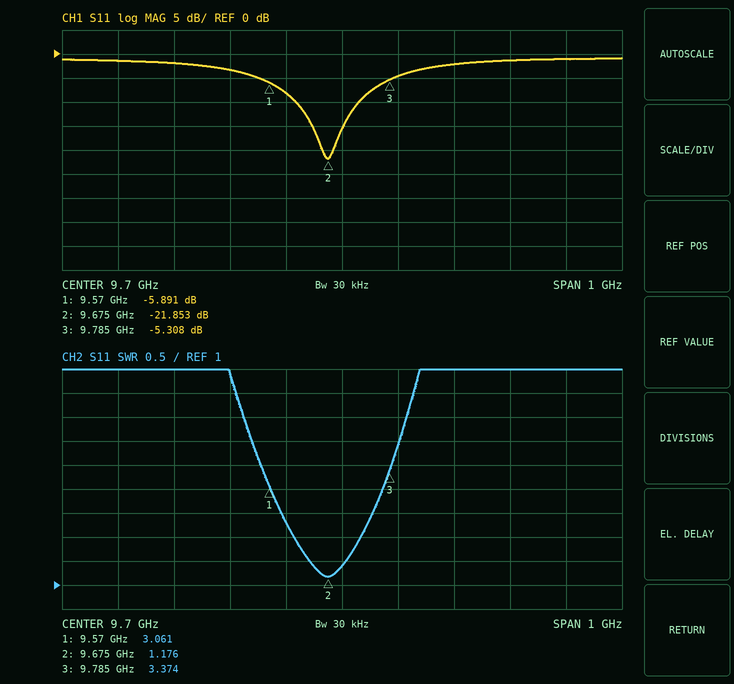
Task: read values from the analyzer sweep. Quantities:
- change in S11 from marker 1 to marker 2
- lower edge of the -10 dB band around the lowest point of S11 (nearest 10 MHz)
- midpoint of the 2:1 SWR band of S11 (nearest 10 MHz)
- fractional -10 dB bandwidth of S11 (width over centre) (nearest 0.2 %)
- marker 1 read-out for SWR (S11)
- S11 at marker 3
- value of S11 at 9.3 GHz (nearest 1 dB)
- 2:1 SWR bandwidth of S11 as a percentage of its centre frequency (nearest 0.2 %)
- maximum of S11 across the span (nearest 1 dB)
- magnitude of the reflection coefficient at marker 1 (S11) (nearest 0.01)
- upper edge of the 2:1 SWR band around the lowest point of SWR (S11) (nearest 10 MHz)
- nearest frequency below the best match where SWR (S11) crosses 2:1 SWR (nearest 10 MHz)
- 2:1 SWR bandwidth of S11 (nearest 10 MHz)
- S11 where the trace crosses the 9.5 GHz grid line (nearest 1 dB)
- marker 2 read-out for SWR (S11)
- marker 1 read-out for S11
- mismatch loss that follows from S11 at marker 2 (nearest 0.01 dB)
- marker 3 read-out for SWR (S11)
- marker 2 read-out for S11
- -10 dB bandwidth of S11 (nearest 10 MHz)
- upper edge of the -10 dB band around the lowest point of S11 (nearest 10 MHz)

-15.962 dB
9.62 GHz
9.67 GHz
1.2 %
3.061
-5.308 dB
-1 dB
1.2 %
-1 dB
0.51
9.73 GHz
9.61 GHz
120 MHz
-3 dB
1.176
-5.891 dB
0.03 dB
3.374
-21.853 dB
110 MHz
9.73 GHz
